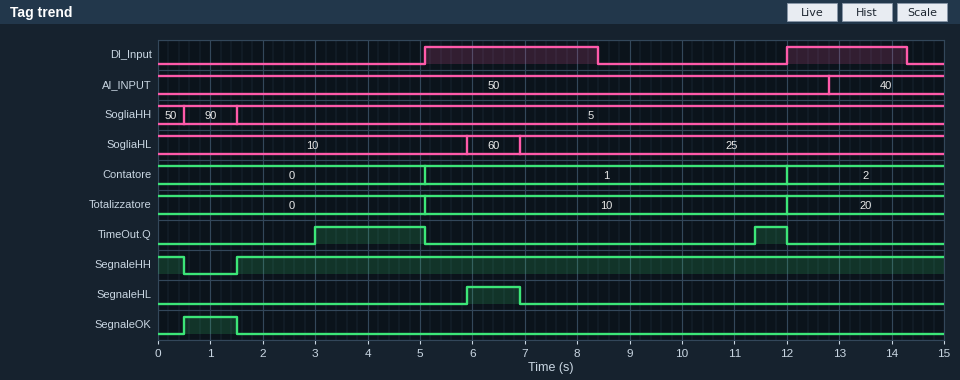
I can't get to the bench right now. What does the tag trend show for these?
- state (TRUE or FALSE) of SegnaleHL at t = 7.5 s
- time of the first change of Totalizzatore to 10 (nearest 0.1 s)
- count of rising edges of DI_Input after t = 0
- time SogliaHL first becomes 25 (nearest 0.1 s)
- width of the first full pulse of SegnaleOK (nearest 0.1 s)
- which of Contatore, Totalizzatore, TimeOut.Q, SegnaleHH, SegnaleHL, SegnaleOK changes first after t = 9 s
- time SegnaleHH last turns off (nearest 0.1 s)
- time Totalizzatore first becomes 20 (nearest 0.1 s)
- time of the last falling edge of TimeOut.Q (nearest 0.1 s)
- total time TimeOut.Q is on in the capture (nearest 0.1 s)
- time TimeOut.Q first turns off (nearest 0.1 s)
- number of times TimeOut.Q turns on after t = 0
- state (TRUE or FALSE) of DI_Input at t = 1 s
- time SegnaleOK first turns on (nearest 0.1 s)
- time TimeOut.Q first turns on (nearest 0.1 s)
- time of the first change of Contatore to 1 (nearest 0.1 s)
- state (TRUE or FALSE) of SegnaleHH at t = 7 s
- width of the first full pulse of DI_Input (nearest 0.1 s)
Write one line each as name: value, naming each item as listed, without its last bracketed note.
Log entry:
state (TRUE or FALSE) of SegnaleHL at t = 7.5 s: FALSE
time of the first change of Totalizzatore to 10: 5.1 s
count of rising edges of DI_Input after t = 0: 2
time SogliaHL first becomes 25: 6.9 s
width of the first full pulse of SegnaleOK: 1.0 s
which of Contatore, Totalizzatore, TimeOut.Q, SegnaleHH, SegnaleHL, SegnaleOK changes first after t = 9 s: TimeOut.Q
time SegnaleHH last turns off: 0.5 s
time Totalizzatore first becomes 20: 12.0 s
time of the last falling edge of TimeOut.Q: 12.0 s
total time TimeOut.Q is on in the capture: 2.7 s
time TimeOut.Q first turns off: 5.1 s
number of times TimeOut.Q turns on after t = 0: 2
state (TRUE or FALSE) of DI_Input at t = 1 s: FALSE
time SegnaleOK first turns on: 0.5 s
time TimeOut.Q first turns on: 3.0 s
time of the first change of Contatore to 1: 5.1 s
state (TRUE or FALSE) of SegnaleHH at t = 7 s: TRUE
width of the first full pulse of DI_Input: 3.3 s
